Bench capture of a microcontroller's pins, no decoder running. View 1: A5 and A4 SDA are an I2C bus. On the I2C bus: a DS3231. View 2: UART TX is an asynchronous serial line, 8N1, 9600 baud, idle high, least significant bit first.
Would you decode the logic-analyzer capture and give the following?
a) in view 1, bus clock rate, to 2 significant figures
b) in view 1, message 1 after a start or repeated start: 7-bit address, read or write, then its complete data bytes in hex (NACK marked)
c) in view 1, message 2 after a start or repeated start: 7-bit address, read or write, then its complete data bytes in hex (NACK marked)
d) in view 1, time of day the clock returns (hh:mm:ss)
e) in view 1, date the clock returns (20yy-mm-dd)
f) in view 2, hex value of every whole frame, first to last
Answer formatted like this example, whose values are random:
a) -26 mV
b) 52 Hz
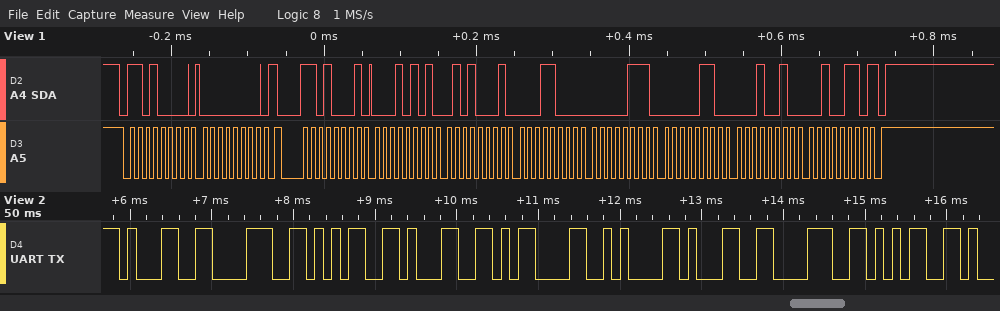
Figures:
a) 100 kHz
b) 0x68 write: 00
c) 0x68 read: 15 51 18 07 06 12 26 NACK
d) 18:51:15
e) 2026-12-06
f) 31 38 35 31 0D 0A 31 38 35
